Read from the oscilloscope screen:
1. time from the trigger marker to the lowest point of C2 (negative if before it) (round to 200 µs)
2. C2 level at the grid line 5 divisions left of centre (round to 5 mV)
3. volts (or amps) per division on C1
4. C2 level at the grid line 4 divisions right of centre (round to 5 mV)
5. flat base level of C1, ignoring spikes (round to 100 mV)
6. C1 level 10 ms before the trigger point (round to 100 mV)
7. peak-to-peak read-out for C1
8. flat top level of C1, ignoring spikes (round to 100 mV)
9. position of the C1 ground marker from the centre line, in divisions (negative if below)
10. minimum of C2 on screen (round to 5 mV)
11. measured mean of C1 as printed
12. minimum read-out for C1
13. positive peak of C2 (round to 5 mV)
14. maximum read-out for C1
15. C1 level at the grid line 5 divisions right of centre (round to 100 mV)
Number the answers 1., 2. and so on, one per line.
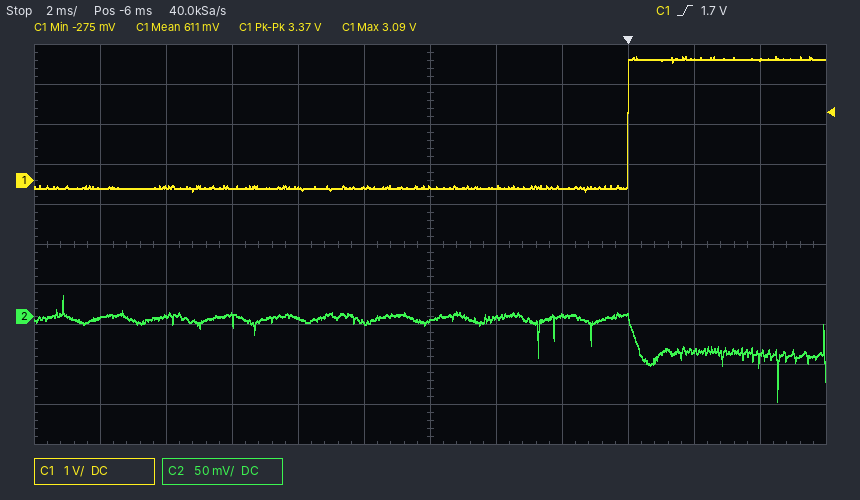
1. +4.6 ms
2. 0 mV
3. 1 V
4. -45 mV
5. -200 mV
6. -200 mV
7. 3.37 V
8. 3.0 V
9. +1.6 div
10. -105 mV
11. 611 mV
12. -275 mV
13. 25 mV
14. 3.09 V
15. 3.0 V
